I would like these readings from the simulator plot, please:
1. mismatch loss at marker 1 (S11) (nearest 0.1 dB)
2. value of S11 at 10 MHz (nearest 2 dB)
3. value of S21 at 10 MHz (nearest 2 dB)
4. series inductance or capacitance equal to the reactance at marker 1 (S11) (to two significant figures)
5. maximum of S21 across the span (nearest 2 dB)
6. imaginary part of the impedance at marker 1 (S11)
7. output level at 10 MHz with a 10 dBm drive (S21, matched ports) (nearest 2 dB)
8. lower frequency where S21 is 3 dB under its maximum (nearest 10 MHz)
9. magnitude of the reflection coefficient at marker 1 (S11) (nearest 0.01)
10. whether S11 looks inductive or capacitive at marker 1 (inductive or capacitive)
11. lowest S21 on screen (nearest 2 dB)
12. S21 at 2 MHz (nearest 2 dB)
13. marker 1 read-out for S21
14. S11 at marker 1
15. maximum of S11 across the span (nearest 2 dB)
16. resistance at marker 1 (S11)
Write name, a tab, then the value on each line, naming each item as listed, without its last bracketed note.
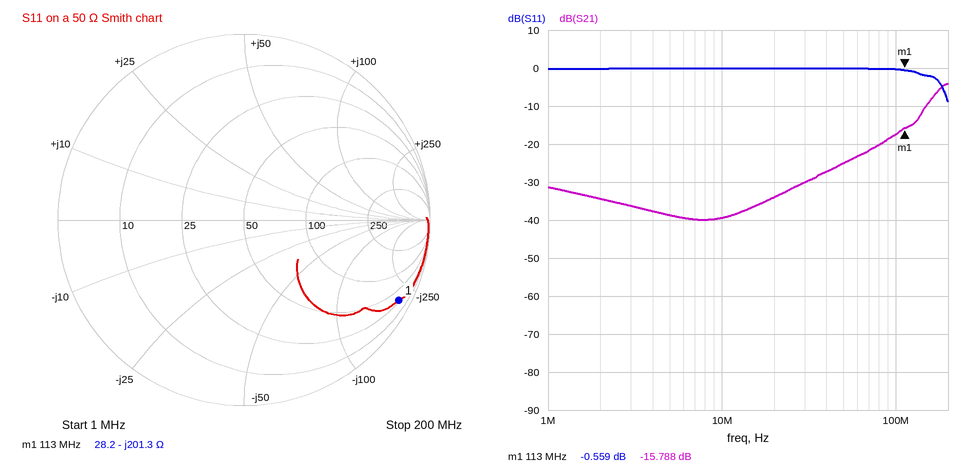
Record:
mismatch loss at marker 1 (S11)	9.2 dB
value of S11 at 10 MHz	0 dB
value of S21 at 10 MHz	-40 dB
series inductance or capacitance equal to the reactance at marker 1 (S11)	7.0 pF
maximum of S21 across the span	-4 dB
imaginary part of the impedance at marker 1	-201.3 Ω
output level at 10 MHz with a 10 dBm drive (S21, matched ports)	-30 dBm
lower frequency where S21 is 3 dB under its maximum	170 MHz
magnitude of the reflection coefficient at marker 1 (S11)	0.94
whether S11 looks inductive or capacitive at marker 1	capacitive
lowest S21 on screen	-40 dB
S21 at 2 MHz	-34 dB
marker 1 read-out for S21	-15.788 dB
S11 at marker 1	-0.559 dB
maximum of S11 across the span	0 dB
resistance at marker 1	28.2 Ω
